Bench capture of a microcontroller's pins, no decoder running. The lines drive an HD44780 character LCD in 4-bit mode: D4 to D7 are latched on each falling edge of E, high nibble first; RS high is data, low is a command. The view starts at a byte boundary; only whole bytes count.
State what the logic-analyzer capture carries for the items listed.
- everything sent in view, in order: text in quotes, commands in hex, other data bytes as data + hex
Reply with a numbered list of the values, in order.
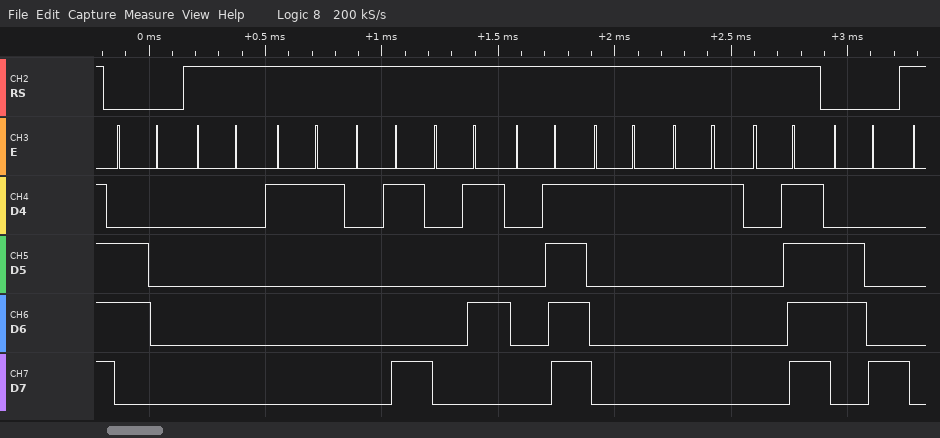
1. 0x60 data 00 11 09 05 0F 11 11 0F 0x68
